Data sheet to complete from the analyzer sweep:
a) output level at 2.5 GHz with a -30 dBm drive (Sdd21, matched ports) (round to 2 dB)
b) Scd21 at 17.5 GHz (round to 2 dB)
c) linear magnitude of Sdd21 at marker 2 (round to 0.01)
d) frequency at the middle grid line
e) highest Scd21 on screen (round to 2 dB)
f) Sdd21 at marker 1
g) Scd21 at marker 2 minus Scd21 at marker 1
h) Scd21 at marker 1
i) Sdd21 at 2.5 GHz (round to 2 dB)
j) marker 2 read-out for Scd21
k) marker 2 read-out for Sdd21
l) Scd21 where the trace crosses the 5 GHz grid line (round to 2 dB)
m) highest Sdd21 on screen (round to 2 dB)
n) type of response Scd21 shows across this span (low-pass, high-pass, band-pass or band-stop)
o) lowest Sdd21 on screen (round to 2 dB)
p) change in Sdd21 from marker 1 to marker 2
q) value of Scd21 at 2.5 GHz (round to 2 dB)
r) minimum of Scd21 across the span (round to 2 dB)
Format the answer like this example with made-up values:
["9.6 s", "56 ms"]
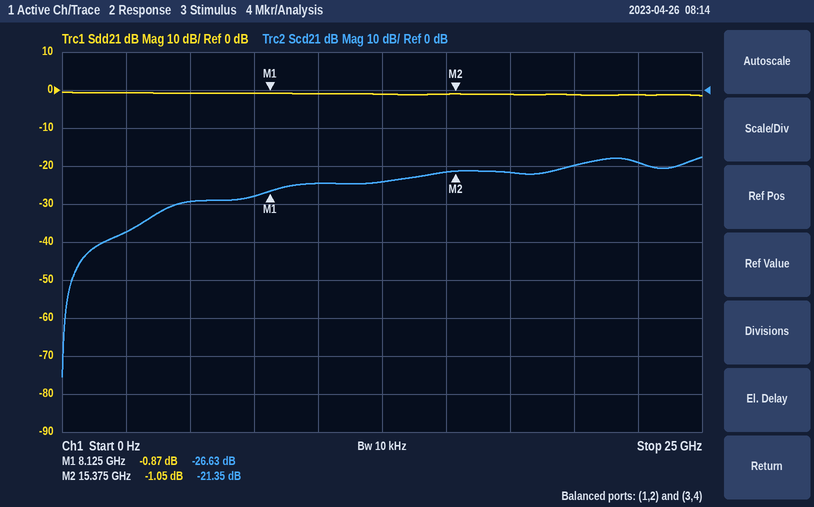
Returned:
["-30 dBm", "-22 dB", "0.89", "12.5 GHz", "-18 dB", "-0.87 dB", "5.28 dB", "-26.63 dB", "0 dB", "-21.35 dB", "-1.05 dB", "-30 dB", "0 dB", "high-pass", "-2 dB", "-0.18 dB", "-38 dB", "-76 dB"]
